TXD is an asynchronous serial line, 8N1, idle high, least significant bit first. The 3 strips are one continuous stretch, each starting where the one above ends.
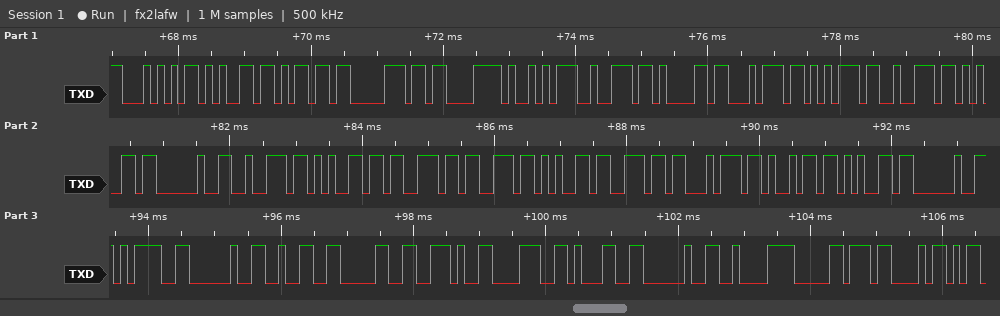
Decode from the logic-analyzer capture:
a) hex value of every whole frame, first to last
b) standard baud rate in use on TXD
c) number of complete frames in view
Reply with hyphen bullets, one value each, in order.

- 0x54 0x65 0x6D 0x70 0xC3 0xA9 0x72 0x61 0x74 0x75 0x72 0x65 0x20 0x72 0x65 0x73 0x73 0x65 0x6E 0x74 0x69 0x65 0x20 0x3D 0x20 0x32 0x30 0x2E 0x38 0x31 0x20 0xC2 0xB0 0x43
- 9600 baud
- 34
